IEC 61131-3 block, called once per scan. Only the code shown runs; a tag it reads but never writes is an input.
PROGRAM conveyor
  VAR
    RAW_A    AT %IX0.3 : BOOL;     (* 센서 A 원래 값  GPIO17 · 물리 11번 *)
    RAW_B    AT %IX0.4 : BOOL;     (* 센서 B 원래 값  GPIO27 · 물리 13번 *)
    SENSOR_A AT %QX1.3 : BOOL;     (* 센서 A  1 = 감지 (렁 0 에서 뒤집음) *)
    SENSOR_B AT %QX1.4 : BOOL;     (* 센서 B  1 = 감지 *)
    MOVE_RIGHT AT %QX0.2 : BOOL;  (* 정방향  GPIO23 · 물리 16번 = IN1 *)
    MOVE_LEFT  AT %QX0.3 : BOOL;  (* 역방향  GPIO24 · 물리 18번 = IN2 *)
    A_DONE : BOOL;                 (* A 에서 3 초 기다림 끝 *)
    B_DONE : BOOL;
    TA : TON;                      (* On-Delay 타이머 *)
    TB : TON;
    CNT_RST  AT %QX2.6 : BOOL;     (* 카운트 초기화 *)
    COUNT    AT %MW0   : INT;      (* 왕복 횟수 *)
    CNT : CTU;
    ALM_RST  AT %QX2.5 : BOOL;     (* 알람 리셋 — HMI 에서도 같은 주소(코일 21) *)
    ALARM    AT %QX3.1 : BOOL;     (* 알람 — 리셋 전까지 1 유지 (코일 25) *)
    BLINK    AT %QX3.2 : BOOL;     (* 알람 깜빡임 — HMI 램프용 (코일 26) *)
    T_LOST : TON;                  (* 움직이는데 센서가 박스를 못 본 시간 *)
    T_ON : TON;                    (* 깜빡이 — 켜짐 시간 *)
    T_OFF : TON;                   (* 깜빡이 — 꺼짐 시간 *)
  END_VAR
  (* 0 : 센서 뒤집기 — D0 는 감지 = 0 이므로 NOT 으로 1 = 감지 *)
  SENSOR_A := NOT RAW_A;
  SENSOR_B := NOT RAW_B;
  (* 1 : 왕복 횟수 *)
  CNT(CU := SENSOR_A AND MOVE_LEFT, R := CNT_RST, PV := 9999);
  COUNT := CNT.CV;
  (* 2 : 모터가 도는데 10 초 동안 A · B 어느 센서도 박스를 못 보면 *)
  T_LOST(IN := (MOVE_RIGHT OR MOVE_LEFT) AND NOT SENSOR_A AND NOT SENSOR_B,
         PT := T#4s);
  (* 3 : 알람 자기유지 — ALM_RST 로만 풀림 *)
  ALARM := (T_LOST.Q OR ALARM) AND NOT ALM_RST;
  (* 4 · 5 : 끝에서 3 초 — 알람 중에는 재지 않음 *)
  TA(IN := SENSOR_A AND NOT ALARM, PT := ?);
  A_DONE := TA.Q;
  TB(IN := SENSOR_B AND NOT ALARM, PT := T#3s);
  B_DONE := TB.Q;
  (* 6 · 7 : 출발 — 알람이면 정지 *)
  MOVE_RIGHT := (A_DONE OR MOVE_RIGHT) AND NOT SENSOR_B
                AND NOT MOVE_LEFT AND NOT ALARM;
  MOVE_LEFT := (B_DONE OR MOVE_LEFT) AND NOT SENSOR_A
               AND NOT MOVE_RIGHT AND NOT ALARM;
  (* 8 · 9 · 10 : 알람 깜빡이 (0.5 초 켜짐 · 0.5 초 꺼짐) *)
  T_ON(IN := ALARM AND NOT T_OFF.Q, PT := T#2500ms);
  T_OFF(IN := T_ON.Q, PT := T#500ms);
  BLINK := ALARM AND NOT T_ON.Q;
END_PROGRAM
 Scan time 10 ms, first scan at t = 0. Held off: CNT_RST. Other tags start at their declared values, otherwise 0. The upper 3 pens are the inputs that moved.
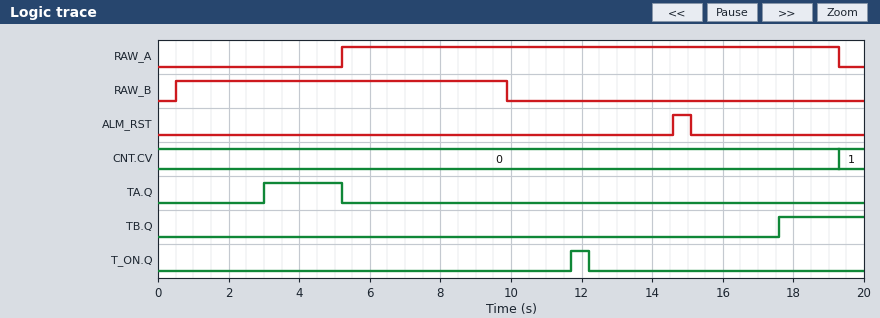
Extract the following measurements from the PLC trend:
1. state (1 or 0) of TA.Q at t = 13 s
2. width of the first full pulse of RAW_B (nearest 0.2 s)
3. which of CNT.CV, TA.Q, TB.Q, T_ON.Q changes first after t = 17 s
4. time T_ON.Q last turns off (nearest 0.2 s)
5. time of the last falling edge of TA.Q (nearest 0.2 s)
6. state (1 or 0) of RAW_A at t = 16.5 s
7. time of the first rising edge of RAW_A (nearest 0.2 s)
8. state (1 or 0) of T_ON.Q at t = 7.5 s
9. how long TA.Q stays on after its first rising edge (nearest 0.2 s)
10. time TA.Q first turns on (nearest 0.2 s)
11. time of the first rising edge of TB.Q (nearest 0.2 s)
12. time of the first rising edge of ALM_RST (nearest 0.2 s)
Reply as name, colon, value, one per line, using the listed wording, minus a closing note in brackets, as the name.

state (1 or 0) of TA.Q at t = 13 s: 0
width of the first full pulse of RAW_B: 9.4 s
which of CNT.CV, TA.Q, TB.Q, T_ON.Q changes first after t = 17 s: TB.Q
time T_ON.Q last turns off: 12.2 s
time of the last falling edge of TA.Q: 5.2 s
state (1 or 0) of RAW_A at t = 16.5 s: 1
time of the first rising edge of RAW_A: 5.2 s
state (1 or 0) of T_ON.Q at t = 7.5 s: 0
how long TA.Q stays on after its first rising edge: 2.2 s
time TA.Q first turns on: 3.0 s
time of the first rising edge of TB.Q: 17.6 s
time of the first rising edge of ALM_RST: 14.6 s
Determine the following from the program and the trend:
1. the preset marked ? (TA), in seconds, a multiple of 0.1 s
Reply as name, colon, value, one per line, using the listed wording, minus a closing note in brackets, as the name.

the preset marked ? (TA), in seconds, a multiple of 0.1 s: 3.0 s
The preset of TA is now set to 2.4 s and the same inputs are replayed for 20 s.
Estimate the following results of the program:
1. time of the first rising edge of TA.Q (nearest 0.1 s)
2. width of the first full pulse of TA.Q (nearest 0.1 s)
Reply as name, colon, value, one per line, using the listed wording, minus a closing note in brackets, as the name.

time of the first rising edge of TA.Q: 2.4 s
width of the first full pulse of TA.Q: 2.8 s
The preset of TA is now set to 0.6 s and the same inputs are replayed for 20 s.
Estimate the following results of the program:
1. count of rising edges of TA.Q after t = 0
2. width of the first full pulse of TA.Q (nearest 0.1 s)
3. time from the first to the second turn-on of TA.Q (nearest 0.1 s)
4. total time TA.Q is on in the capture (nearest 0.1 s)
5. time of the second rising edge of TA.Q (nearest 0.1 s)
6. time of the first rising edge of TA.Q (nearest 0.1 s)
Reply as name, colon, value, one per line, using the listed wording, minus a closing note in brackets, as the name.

count of rising edges of TA.Q after t = 0: 2
width of the first full pulse of TA.Q: 4.6 s
time from the first to the second turn-on of TA.Q: 19.3 s
total time TA.Q is on in the capture: 4.7 s
time of the second rising edge of TA.Q: 19.9 s
time of the first rising edge of TA.Q: 0.6 s
